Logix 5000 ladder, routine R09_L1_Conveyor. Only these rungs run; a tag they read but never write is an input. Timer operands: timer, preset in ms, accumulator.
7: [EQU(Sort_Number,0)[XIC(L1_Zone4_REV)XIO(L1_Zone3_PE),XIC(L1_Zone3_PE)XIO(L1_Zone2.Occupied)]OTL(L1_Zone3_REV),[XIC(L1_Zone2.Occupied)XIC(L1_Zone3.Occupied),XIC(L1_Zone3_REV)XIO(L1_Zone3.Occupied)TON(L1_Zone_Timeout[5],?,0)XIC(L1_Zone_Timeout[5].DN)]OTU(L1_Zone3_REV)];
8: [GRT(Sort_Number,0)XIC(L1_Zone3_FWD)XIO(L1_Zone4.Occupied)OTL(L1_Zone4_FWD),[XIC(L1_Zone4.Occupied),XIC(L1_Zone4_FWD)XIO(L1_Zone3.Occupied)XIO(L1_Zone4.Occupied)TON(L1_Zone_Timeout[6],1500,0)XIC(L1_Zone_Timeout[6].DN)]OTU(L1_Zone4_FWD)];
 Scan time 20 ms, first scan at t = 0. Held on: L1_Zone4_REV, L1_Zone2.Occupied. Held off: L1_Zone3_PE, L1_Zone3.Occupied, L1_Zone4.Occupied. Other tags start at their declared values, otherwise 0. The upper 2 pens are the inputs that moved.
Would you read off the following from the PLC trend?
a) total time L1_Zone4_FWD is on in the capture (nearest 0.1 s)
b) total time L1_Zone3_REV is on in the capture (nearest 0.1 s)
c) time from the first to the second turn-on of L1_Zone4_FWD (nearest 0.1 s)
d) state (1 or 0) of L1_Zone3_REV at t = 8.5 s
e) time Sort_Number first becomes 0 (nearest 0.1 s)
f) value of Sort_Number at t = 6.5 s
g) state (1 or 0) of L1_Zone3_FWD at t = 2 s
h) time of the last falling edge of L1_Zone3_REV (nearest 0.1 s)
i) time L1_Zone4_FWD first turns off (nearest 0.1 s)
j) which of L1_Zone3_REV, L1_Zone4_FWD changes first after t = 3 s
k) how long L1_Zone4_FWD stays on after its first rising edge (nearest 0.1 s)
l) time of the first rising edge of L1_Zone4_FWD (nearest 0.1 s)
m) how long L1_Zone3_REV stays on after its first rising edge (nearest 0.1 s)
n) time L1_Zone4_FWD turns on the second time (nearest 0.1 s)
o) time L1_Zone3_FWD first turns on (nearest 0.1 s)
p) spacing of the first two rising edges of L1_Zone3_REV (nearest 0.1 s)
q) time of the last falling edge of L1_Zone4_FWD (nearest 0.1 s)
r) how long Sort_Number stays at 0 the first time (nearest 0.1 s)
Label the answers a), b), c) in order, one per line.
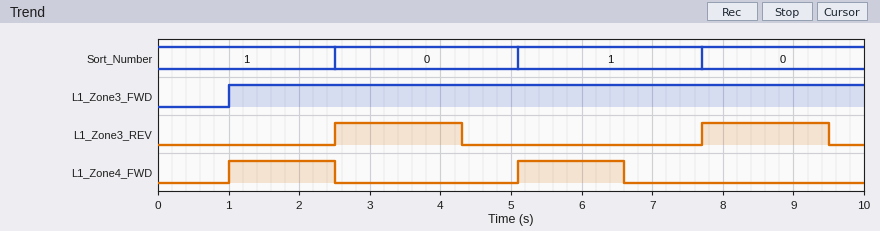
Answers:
a) 3.0 s
b) 3.6 s
c) 4.1 s
d) 1
e) 2.5 s
f) 1
g) 1
h) 9.5 s
i) 2.5 s
j) L1_Zone3_REV
k) 1.5 s
l) 1.0 s
m) 1.8 s
n) 5.1 s
o) 1.0 s
p) 5.2 s
q) 6.6 s
r) 2.6 s
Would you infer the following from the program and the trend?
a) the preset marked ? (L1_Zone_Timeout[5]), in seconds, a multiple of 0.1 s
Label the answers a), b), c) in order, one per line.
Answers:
a) 1.8 s
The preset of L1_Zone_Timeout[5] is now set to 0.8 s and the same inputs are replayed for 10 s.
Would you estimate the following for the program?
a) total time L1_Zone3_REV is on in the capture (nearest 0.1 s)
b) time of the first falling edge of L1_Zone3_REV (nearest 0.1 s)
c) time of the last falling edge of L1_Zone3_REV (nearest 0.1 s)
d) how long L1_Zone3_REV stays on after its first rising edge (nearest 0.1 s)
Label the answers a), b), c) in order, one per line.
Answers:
a) 1.6 s
b) 3.3 s
c) 8.5 s
d) 0.8 s
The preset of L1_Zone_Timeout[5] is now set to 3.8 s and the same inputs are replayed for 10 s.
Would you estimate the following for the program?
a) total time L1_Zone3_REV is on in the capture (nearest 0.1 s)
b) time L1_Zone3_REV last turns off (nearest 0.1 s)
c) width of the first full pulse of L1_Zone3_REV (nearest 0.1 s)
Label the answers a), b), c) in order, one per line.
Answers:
a) 6.1 s
b) 6.3 s
c) 3.8 s
